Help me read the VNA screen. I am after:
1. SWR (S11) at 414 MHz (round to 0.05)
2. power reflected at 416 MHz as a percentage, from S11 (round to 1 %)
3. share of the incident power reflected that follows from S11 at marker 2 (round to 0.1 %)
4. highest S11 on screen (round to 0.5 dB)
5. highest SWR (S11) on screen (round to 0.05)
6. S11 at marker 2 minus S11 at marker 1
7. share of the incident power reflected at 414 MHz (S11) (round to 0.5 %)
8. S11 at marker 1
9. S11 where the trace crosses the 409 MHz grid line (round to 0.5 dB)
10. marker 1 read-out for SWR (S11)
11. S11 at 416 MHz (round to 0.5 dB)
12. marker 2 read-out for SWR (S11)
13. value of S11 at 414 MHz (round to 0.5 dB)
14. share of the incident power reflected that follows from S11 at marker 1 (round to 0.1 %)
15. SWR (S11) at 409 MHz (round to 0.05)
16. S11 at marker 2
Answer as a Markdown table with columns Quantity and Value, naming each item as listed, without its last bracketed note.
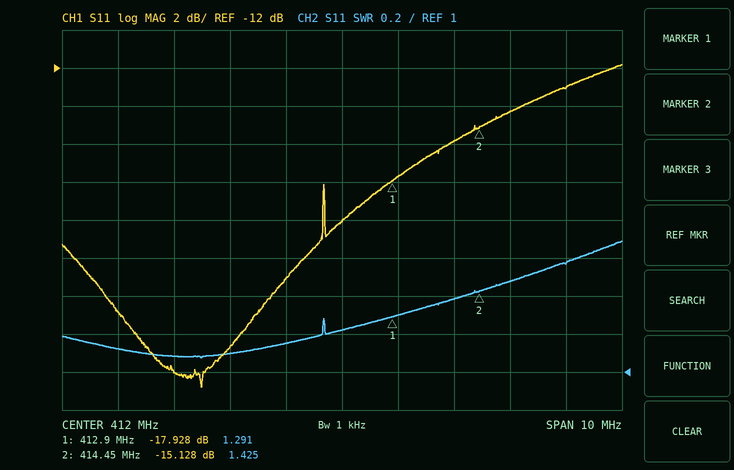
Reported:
| Quantity | Value |
|---|---|
| SWR (S11) at 414 MHz | 1.40 |
| power reflected at 416 MHz as a percentage, from S11 | 5 % |
| share of the incident power reflected that follows from S11 at marker 2 | 3.1 % |
| highest S11 on screen | -12.0 dB |
| highest SWR (S11) on screen | 1.70 |
| S11 at marker 2 minus S11 at marker 1 | 2.800 dB |
| share of the incident power reflected at 414 MHz (S11) | 2.5 % |
| S11 at marker 1 | -17.928 dB |
| S11 where the trace crosses the 409 MHz grid line | -28.0 dB |
| marker 1 read-out for SWR | 1.291 |
| S11 at 416 MHz | -13.0 dB |
| marker 2 read-out for SWR | 1.425 |
| value of S11 at 414 MHz | -16.0 dB |
| share of the incident power reflected that follows from S11 at marker 1 | 1.6 % |
| SWR (S11) at 409 MHz | 1.10 |
| S11 at marker 2 | -15.128 dB |
